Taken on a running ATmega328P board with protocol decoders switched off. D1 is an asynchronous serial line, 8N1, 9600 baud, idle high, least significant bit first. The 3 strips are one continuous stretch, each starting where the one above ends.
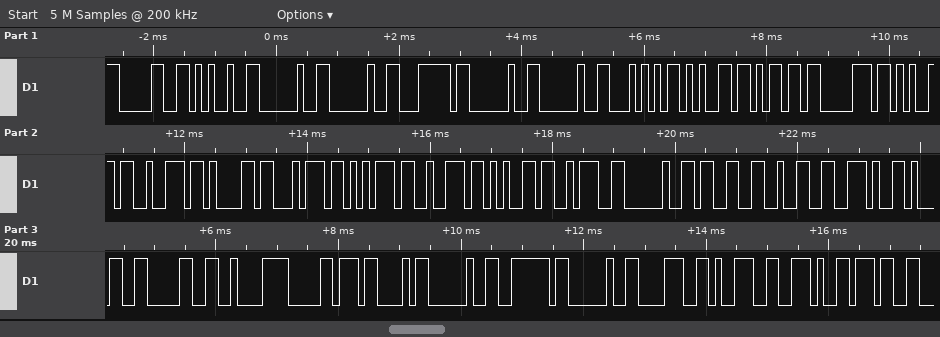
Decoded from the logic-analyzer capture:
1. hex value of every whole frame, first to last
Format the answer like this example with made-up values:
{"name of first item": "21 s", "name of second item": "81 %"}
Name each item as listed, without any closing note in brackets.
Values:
{"hex value of every whole frame, first to last": "30 25 20 20 7C 20 20 54 65 6D 70 65 72 61 74 75 72 65 3A 20 33 32 2E 31 30 C2 B0 43 20 7E 20 38 39 2E 37"}
